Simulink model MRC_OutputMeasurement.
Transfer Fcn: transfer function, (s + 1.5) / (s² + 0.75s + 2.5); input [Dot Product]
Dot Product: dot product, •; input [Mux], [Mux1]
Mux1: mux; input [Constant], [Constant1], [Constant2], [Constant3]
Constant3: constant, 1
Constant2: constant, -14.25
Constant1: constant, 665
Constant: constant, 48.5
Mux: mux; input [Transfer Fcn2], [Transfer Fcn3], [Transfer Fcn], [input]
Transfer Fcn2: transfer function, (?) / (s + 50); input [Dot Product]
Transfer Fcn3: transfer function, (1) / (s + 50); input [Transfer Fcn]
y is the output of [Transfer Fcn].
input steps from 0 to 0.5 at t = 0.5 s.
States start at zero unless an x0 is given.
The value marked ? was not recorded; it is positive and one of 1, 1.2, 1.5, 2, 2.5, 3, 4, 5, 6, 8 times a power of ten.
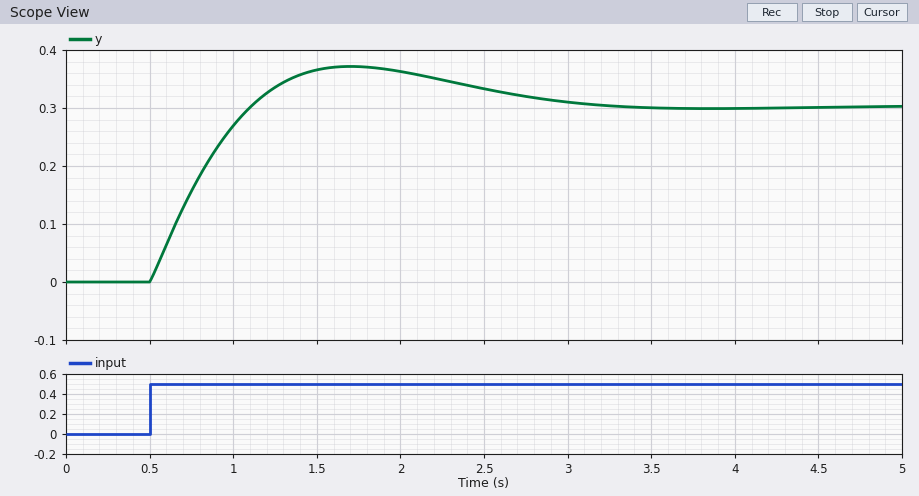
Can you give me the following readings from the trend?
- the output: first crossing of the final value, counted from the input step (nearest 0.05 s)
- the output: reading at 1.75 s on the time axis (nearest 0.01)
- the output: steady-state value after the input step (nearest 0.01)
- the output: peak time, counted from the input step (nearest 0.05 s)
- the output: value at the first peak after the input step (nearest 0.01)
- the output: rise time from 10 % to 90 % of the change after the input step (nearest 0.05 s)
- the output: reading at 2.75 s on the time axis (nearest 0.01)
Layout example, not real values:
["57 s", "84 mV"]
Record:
["0.60 s", "0.37", "0.30", "1.20 s", "0.37", "0.45 s", "0.32"]
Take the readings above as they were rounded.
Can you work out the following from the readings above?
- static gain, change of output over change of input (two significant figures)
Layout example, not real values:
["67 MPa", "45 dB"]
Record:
["0.60"]
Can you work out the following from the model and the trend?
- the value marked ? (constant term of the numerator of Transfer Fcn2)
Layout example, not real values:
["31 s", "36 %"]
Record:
["0.6"]
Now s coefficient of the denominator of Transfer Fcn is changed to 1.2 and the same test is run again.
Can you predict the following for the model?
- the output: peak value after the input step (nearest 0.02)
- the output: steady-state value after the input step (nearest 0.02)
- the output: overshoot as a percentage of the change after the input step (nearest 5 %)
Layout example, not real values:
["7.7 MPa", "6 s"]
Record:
["0.36", "0.30", "15 %"]
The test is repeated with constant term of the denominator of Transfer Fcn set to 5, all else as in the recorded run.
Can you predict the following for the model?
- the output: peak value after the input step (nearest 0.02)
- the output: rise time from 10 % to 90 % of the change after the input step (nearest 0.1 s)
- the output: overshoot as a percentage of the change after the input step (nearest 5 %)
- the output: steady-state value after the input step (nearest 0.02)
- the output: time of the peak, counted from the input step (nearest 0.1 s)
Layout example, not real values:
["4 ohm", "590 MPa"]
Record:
["0.30", "0.3 s", "40 %", "0.22", "0.9 s"]
